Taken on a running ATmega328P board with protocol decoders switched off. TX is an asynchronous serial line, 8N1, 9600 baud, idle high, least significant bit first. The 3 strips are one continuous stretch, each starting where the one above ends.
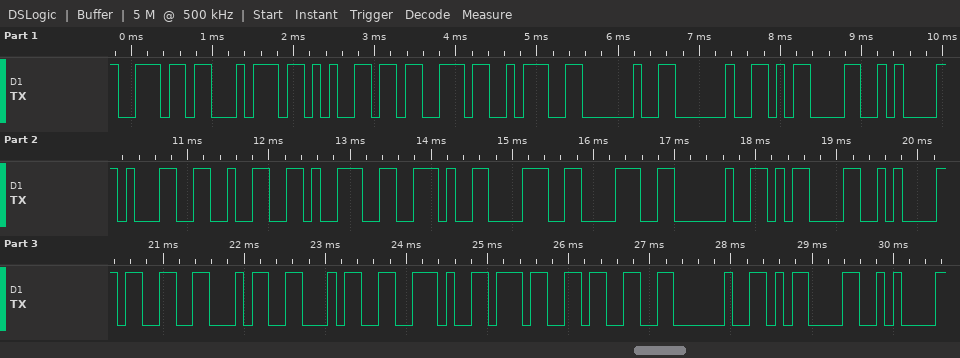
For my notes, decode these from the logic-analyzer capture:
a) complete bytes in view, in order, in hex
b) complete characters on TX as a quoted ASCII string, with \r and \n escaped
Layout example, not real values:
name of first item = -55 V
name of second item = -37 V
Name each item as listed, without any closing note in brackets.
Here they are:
complete bytes in view, in order, in hex = 6E 74 65 73 3A 20 20 0D 0A 31 32 39 2E 38 38 20 0D 0A 33 34 34 2E 37 33 20 0D 0A
complete characters on TX as a quoted ASCII string, with \r and \n escaped = "ntes:  \r\n129.88 \r\n344.73 \r\n"
